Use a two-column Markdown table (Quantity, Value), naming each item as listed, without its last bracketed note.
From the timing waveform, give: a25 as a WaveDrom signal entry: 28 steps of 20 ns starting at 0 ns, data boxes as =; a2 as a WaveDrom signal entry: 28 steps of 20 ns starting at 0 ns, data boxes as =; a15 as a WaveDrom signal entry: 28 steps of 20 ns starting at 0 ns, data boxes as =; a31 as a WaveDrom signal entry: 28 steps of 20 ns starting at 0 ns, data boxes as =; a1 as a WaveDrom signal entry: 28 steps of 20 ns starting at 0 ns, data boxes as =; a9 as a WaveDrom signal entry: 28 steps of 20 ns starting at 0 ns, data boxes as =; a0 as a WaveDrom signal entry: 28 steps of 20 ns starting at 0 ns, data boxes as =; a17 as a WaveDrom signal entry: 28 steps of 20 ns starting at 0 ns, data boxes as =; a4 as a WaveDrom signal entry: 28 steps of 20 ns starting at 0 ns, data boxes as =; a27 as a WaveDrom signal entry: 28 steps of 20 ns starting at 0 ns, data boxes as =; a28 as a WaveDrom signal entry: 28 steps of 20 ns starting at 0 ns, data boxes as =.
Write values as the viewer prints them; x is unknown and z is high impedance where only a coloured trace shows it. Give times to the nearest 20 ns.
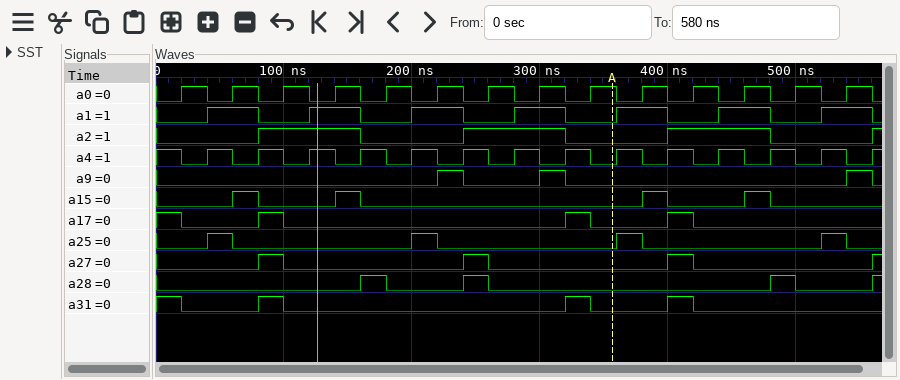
| Quantity | Value |
|---|---|
| a25 as a WaveDrom signal entry: 28 steps of 20 ns starting at 0 ns, data boxes as = | {name: 'a25', wave: '0.10......10......10......10'} |
| a2 as a WaveDrom signal entry: 28 steps of 20 ns starting at 0 ns, data boxes as = | {name: 'a2', wave: '0...1...0...1...0...1...0...'} |
| a15 as a WaveDrom signal entry: 28 steps of 20 ns starting at 0 ns, data boxes as = | {name: 'a15', wave: '0..10..10..........10..10...'} |
| a31 as a WaveDrom signal entry: 28 steps of 20 ns starting at 0 ns, data boxes as = | {name: 'a31', wave: '10..10..........10..10......'} |
| a1 as a WaveDrom signal entry: 28 steps of 20 ns starting at 0 ns, data boxes as = | {name: 'a1', wave: '0.1.0.1.0.1.0.1.0.1.0.1.0.1.'} |
| a9 as a WaveDrom signal entry: 28 steps of 20 ns starting at 0 ns, data boxes as = | {name: 'a9', wave: '0..........10..10..........1'} |
| a0 as a WaveDrom signal entry: 28 steps of 20 ns starting at 0 ns, data boxes as = | {name: 'a0', wave: '0101010101010101010101010101'} |
| a17 as a WaveDrom signal entry: 28 steps of 20 ns starting at 0 ns, data boxes as = | {name: 'a17', wave: '10..10..........10..10......'} |
| a4 as a WaveDrom signal entry: 28 steps of 20 ns starting at 0 ns, data boxes as = | {name: 'a4', wave: '1010101010101010101010101010'} |
| a27 as a WaveDrom signal entry: 28 steps of 20 ns starting at 0 ns, data boxes as = | {name: 'a27', wave: '0...10......10......10......'} |
| a28 as a WaveDrom signal entry: 28 steps of 20 ns starting at 0 ns, data boxes as = | {name: 'a28', wave: '0.......10..10..........10..'} |
